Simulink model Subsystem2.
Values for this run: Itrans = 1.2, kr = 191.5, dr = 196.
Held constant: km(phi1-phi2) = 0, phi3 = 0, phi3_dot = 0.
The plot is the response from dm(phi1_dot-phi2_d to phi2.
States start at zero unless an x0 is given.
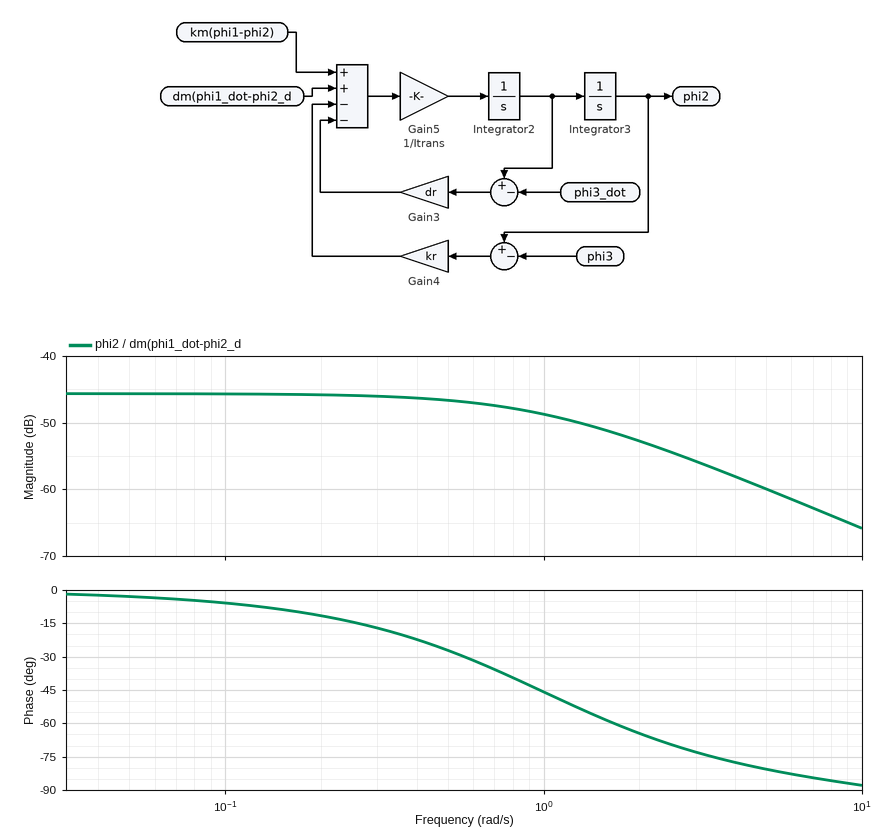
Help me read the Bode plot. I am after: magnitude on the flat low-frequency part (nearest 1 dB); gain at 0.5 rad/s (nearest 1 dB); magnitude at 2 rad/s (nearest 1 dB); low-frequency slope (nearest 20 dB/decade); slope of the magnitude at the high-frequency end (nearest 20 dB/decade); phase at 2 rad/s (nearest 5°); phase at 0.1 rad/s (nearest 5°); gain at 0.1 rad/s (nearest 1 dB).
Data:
-46 dB
-47 dB
-53 dB
0 dB/decade
-20 dB/decade
-65°
-5°
-46 dB
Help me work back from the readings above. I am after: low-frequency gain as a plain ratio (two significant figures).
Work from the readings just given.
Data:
0.0050
